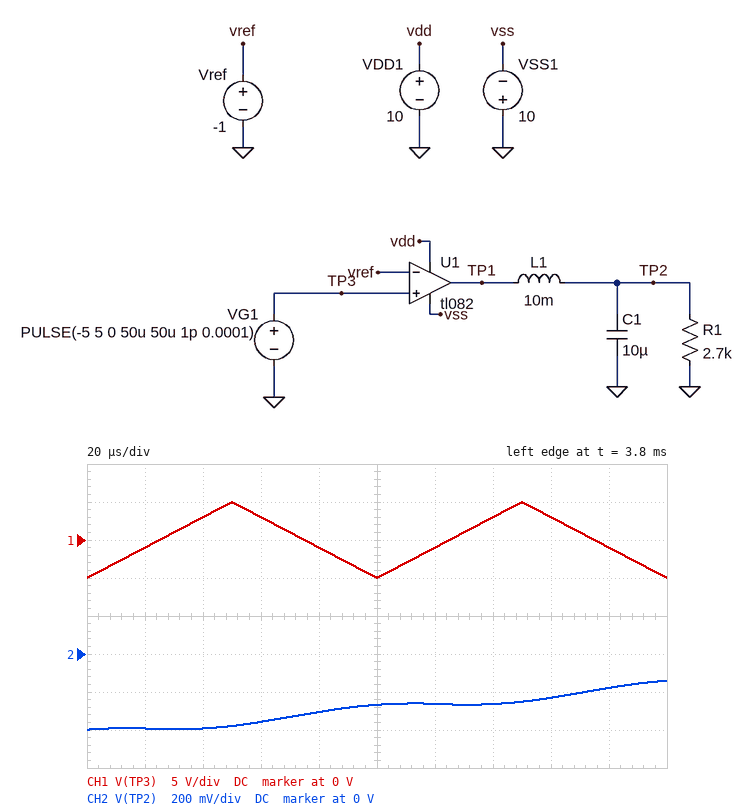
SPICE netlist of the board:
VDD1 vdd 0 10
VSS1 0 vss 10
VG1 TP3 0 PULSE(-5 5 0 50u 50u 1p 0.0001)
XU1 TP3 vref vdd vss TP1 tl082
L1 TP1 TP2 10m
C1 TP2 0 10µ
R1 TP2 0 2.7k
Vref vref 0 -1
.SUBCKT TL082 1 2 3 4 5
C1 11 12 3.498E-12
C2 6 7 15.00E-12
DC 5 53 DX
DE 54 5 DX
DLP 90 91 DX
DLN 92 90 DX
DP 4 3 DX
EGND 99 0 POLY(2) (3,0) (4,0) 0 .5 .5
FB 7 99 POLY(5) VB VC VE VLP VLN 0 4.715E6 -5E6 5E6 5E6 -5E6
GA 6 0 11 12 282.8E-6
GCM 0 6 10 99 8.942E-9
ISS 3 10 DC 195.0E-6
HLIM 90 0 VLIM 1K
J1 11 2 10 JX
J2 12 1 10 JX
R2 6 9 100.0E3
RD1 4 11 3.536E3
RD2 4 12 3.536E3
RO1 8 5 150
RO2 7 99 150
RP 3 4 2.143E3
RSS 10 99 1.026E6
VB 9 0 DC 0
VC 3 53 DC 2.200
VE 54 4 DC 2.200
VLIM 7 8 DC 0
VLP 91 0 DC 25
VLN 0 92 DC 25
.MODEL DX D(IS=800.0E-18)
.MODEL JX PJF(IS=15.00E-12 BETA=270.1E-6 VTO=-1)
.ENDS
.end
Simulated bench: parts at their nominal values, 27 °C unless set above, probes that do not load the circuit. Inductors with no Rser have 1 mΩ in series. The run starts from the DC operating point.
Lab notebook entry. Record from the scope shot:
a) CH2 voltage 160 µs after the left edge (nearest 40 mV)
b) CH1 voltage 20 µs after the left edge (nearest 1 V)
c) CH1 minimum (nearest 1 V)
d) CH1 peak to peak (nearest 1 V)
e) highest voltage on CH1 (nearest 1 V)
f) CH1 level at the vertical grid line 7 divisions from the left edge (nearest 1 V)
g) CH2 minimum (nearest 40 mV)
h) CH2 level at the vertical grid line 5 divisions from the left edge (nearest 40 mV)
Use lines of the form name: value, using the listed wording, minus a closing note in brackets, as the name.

CH2 voltage 160 µs after the left edge: -240 mV
CH1 voltage 20 µs after the left edge: -1 V
CH1 minimum: -5 V
CH1 peak to peak: 10 V
highest voltage on CH1: 5 V
CH1 level at the vertical grid line 7 divisions from the left edge: 3 V
CH2 minimum: -400 mV
CH2 level at the vertical grid line 5 divisions from the left edge: -280 mV
